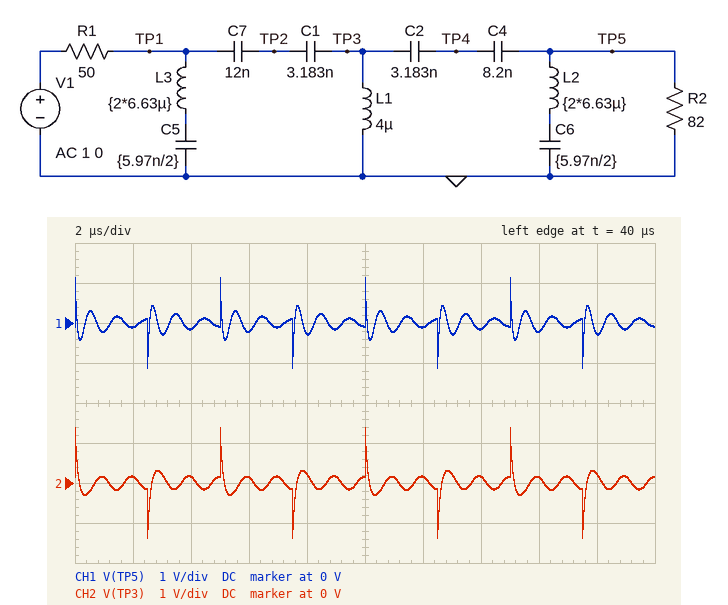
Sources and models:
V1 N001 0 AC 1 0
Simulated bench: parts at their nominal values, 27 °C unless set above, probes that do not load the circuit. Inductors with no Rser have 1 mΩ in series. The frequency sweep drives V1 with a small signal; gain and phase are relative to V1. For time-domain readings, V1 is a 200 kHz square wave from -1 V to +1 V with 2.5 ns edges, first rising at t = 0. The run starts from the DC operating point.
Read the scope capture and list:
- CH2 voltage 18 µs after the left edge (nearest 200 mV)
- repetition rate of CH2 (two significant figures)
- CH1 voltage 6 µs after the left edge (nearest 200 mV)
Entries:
200 mV
200 kHz
-200 mV
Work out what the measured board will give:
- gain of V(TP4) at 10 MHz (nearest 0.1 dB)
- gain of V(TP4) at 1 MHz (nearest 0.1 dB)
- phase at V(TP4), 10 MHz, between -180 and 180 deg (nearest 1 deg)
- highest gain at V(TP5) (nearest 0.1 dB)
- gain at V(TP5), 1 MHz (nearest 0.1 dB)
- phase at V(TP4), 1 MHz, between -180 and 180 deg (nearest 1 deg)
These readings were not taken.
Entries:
-4.2 dB
-12.0 dB
16 deg
-4.0 dB
-4.5 dB
-135 deg
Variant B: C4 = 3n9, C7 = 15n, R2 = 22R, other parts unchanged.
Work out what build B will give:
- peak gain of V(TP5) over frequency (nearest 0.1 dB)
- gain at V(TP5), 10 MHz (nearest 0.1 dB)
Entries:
-10.1 dB
-10.3 dB
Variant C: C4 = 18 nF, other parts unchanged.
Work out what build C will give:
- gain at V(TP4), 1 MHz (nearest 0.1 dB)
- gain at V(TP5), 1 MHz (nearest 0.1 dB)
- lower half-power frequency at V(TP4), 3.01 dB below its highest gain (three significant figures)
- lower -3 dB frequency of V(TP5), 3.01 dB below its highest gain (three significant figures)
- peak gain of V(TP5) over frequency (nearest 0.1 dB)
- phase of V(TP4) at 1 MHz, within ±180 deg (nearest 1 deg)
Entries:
-8.5 dB
-5.6 dB
1.06 MHz
916 kHz
-3.9 dB
-128 deg
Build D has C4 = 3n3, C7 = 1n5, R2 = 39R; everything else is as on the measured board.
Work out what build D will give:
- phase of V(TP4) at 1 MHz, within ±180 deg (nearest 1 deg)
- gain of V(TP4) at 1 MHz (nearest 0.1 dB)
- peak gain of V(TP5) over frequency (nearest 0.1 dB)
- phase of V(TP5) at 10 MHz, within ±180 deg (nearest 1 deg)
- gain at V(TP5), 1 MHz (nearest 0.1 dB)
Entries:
-119 deg
-22.4 dB
-7.2 dB
24 deg
-25.2 dB
